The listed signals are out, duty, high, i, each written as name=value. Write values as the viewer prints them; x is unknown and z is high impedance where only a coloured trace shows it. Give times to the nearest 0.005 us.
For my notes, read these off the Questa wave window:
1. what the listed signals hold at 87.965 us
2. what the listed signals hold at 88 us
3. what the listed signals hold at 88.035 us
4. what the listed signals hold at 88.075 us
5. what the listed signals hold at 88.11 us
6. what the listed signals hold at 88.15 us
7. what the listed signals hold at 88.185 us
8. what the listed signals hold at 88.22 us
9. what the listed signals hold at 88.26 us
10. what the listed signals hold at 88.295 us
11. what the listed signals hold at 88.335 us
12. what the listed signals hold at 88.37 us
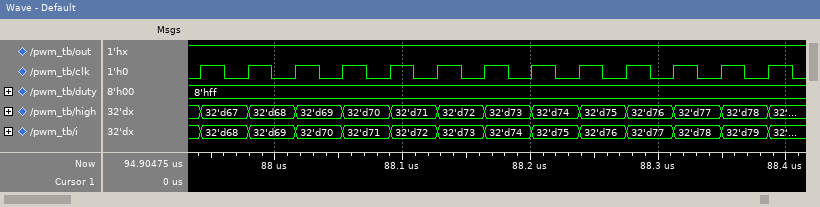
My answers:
out=1, duty=8'hff, high=32'd67, i=32'd68
out=1, duty=8'hff, high=32'd68, i=32'd69
out=1, duty=8'hff, high=32'd69, i=32'd70
out=1, duty=8'hff, high=32'd70, i=32'd71
out=1, duty=8'hff, high=32'd71, i=32'd72
out=1, duty=8'hff, high=32'd72, i=32'd73
out=1, duty=8'hff, high=32'd73, i=32'd74
out=1, duty=8'hff, high=32'd74, i=32'd75
out=1, duty=8'hff, high=32'd75, i=32'd76
out=1, duty=8'hff, high=32'd76, i=32'd77
out=1, duty=8'hff, high=32'd77, i=32'd78
out=1, duty=8'hff, high=32'd78, i=32'd79
